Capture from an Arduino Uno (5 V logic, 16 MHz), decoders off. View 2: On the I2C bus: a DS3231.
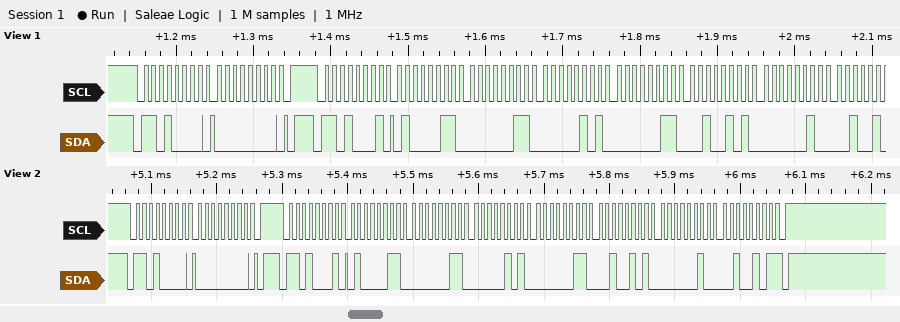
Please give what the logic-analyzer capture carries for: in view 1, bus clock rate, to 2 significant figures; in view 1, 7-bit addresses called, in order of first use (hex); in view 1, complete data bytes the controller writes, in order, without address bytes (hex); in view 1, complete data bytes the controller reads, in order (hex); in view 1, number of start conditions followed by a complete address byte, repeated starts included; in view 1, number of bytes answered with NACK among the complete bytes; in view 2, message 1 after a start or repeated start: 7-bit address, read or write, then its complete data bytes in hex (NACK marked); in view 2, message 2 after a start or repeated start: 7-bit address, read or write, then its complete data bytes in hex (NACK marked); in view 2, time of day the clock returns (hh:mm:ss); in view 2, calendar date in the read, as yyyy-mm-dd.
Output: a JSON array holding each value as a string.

["100 kHz", "0x68", "00", "43 03 05 03 25 02", "2", "0", "0x68 write: 00", "0x68 read: 43 03 05 03 25 02 25 NACK", "05:03:43", "2025-02-25"]
